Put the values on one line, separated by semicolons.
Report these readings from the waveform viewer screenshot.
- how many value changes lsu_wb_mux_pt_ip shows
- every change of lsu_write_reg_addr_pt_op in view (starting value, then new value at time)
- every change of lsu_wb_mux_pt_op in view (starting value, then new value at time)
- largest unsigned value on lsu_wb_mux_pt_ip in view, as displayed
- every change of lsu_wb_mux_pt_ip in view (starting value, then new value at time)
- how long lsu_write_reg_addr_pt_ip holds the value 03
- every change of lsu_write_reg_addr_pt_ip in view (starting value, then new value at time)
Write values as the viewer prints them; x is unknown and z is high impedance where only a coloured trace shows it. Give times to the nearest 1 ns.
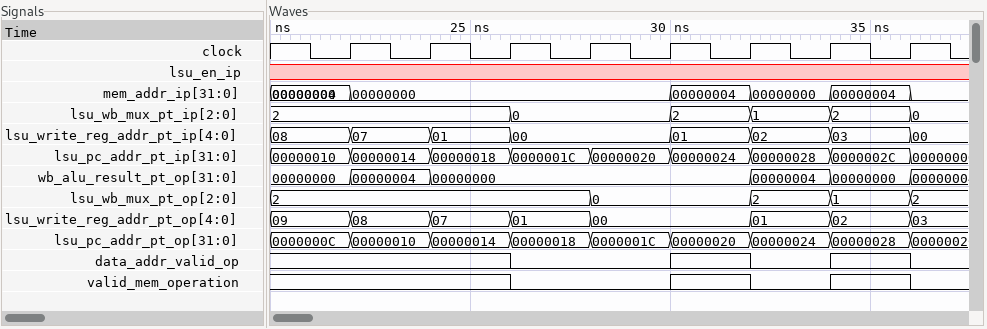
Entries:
5; 09, 08 at 22 ns, 07 at 24 ns, 01 at 26 ns, 00 at 28 ns, 01 at 32 ns, 02 at 34 ns, 03 at 36 ns; 2, 0 at 28 ns, 2 at 32 ns, 1 at 34 ns, 2 at 36 ns; 2; 2, 0 at 26 ns, 2 at 30 ns, 1 at 32 ns, 2 at 34 ns, 0 at 36 ns; 2 ns; 08, 07 at 22 ns, 01 at 24 ns, 00 at 26 ns, 01 at 30 ns, 02 at 32 ns, 03 at 34 ns, 00 at 36 ns
